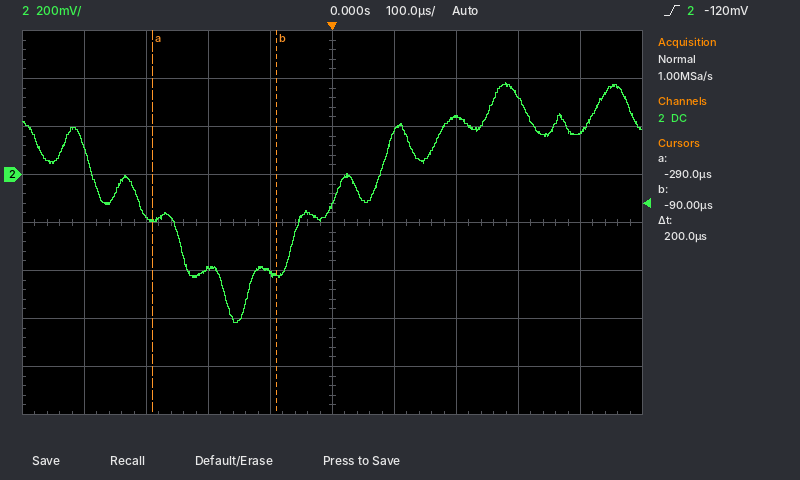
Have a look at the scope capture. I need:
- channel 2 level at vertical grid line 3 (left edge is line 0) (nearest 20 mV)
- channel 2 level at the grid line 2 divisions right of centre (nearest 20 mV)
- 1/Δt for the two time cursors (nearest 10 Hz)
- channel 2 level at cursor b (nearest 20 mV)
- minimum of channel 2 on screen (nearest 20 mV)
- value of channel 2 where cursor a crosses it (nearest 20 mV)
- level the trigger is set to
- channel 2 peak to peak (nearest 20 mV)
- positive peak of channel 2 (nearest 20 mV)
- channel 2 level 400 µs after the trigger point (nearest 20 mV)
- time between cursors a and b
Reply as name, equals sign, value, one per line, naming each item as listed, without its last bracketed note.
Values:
channel 2 level at vertical grid line 3 (left edge is line 0) = -400 mV
channel 2 level at the grid line 2 divisions right of centre = 240 mV
1/Δt for the two time cursors = 5.00 kHz
channel 2 level at cursor b = -420 mV
minimum of channel 2 on screen = -620 mV
value of channel 2 where cursor a crosses it = -200 mV
level the trigger is set to = -120 mV
channel 2 peak to peak = 1.00 V
positive peak of channel 2 = 380 mV
channel 2 level 400 µs after the trigger point = 180 mV
time between cursors a and b = 200 µs
